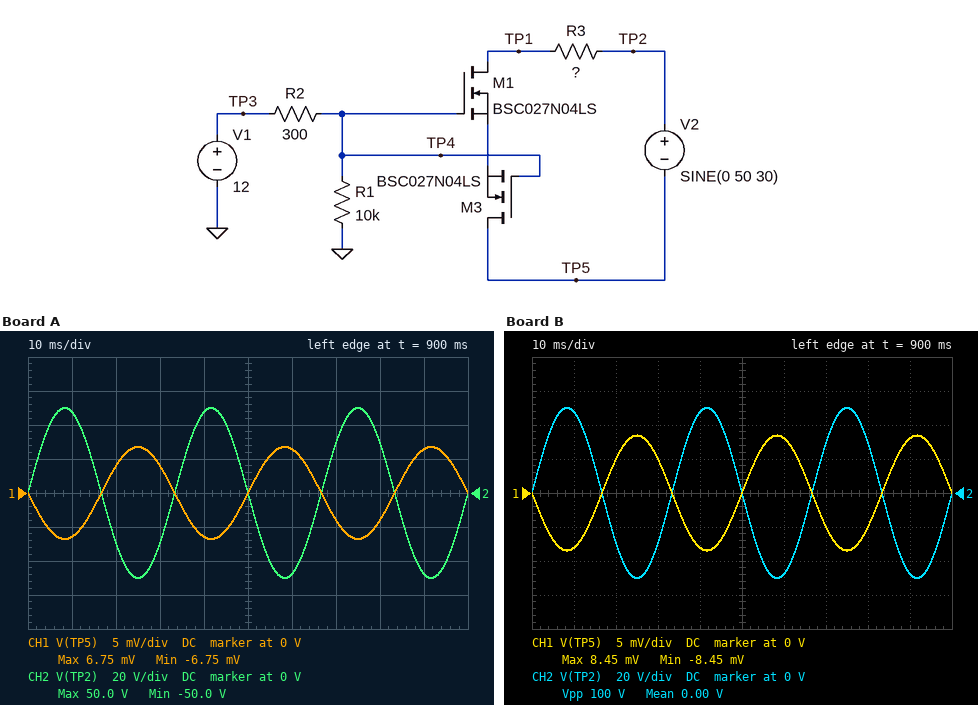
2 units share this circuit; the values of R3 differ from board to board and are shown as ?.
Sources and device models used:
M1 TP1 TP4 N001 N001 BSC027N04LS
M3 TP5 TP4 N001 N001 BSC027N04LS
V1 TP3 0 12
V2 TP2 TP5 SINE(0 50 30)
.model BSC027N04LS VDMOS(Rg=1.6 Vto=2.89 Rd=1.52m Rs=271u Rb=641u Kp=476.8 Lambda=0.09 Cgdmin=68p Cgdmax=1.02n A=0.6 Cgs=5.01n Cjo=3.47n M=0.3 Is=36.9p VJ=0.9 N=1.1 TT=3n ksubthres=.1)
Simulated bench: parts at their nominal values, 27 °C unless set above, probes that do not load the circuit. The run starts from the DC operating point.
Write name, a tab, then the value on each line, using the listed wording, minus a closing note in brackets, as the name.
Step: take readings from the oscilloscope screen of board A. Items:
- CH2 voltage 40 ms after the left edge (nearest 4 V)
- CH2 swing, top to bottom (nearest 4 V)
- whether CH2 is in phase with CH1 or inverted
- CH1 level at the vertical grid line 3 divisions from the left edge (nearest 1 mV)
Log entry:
CH2 voltage 40 ms after the left edge	48 V
CH2 swing, top to bottom	100 V
whether CH2 is in phase with CH1 or inverted	inverted
CH1 level at the vertical grid line 3 divisions from the left edge	4 mV
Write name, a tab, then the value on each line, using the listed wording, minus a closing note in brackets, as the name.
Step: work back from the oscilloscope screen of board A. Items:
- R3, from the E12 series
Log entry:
R3, from the E12 series	15 Ω
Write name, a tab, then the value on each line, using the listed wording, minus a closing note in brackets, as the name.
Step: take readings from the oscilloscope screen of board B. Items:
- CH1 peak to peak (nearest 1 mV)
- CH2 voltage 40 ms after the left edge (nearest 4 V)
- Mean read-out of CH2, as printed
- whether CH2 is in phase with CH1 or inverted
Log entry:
CH1 peak to peak	17 mV
CH2 voltage 40 ms after the left edge	48 V
Mean read-out of CH2, as printed	0.00 V
whether CH2 is in phase with CH1 or inverted	inverted
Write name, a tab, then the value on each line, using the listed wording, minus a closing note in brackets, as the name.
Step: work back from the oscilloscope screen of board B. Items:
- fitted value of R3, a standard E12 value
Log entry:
fitted value of R3, a standard E12 value	12 Ω
